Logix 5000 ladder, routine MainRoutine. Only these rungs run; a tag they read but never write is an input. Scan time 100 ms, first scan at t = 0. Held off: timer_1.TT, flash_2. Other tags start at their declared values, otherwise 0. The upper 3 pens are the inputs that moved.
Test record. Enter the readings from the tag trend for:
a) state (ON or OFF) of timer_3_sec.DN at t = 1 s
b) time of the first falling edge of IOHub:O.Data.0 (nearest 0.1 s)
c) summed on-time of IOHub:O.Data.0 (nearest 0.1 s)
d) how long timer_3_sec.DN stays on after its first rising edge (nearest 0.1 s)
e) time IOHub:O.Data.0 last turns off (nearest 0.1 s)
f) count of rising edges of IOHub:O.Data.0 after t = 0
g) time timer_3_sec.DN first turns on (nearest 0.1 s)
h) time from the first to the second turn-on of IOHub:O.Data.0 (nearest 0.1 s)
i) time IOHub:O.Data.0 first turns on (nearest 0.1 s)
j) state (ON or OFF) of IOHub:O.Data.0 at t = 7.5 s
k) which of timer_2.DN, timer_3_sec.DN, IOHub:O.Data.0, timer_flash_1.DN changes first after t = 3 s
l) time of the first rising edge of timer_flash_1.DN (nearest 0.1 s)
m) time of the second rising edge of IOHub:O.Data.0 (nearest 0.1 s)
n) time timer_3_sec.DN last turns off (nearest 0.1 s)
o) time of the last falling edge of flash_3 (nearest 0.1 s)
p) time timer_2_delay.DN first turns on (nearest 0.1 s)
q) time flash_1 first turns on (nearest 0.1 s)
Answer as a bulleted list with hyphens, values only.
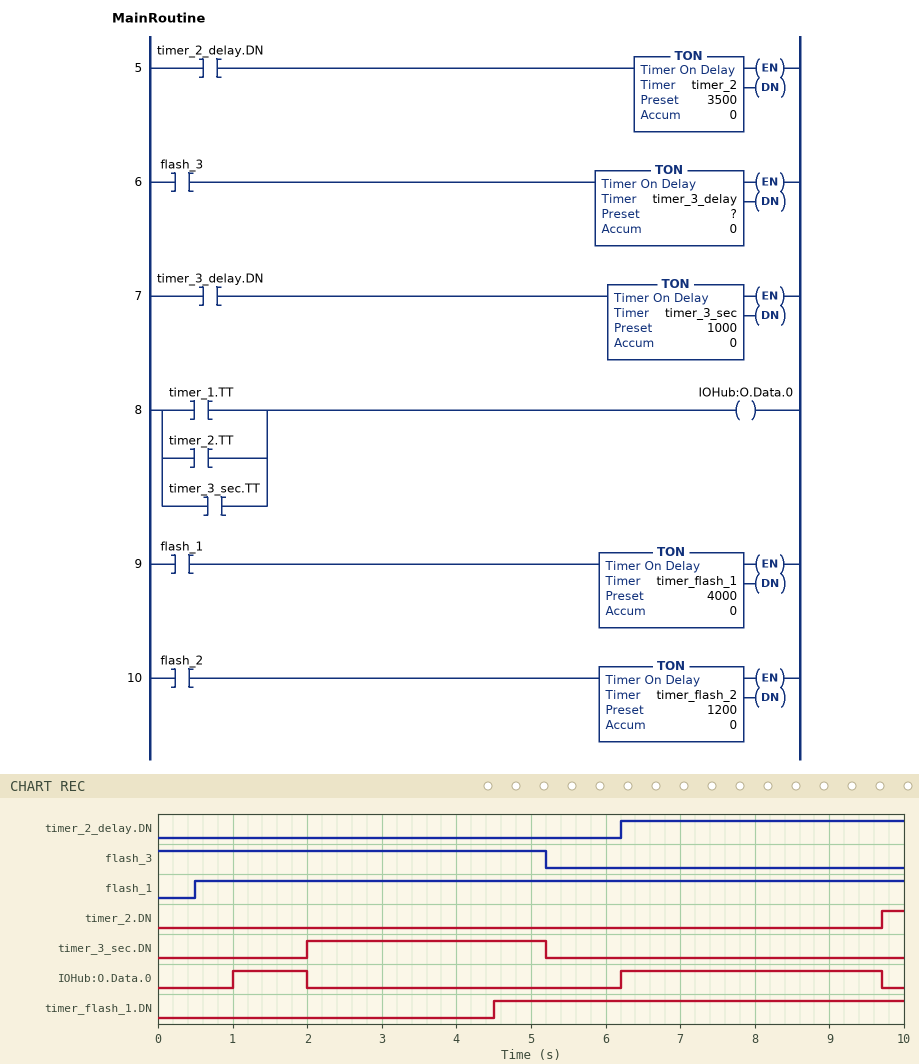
- OFF
- 2.0 s
- 4.5 s
- 3.2 s
- 9.7 s
- 2
- 2.0 s
- 5.2 s
- 1.0 s
- ON
- timer_flash_1.DN
- 4.5 s
- 6.2 s
- 5.2 s
- 5.2 s
- 6.2 s
- 0.5 s
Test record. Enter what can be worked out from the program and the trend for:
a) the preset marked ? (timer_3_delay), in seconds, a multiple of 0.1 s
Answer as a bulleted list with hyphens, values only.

- 1.0 s
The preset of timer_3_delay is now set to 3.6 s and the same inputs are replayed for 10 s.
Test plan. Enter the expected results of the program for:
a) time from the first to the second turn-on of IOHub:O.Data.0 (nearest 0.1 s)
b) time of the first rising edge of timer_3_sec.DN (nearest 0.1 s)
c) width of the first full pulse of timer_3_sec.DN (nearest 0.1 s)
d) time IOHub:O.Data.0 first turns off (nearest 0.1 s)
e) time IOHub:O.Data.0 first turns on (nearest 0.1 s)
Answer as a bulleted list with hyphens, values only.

- 2.6 s
- 4.6 s
- 0.6 s
- 4.6 s
- 3.6 s
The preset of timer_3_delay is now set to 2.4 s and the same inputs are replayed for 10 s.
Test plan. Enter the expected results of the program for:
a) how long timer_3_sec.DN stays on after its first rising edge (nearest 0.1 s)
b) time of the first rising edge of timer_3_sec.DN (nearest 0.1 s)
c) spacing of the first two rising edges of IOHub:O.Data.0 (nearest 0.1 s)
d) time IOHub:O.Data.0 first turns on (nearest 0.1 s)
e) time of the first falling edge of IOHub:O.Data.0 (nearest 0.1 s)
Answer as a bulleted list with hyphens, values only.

- 1.8 s
- 3.4 s
- 3.8 s
- 2.4 s
- 3.4 s
